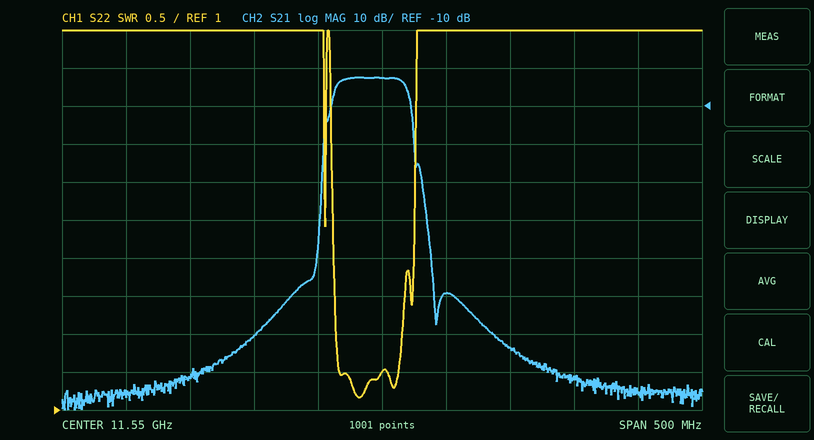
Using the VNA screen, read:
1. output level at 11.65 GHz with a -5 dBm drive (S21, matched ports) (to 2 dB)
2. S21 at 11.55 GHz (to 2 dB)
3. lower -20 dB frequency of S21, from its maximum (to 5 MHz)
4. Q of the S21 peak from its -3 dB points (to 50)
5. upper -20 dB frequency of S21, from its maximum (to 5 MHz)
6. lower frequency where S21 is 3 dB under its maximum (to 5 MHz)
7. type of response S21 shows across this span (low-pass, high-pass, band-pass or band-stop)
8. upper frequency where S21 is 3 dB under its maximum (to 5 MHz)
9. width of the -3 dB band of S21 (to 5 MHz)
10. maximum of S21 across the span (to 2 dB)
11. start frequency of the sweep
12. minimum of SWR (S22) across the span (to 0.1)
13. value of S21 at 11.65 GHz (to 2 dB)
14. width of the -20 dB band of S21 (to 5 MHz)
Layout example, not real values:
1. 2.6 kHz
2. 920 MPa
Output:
1. -78 dBm
2. -2 dB
3. 11.505 GHz
4. 200
5. 11.575 GHz
6. 11.515 GHz
7. band-pass
8. 11.570 GHz
9. 55 MHz
10. -2 dB
11. 11.3 GHz
12. 1.2
13. -74 dB
14. 70 MHz
